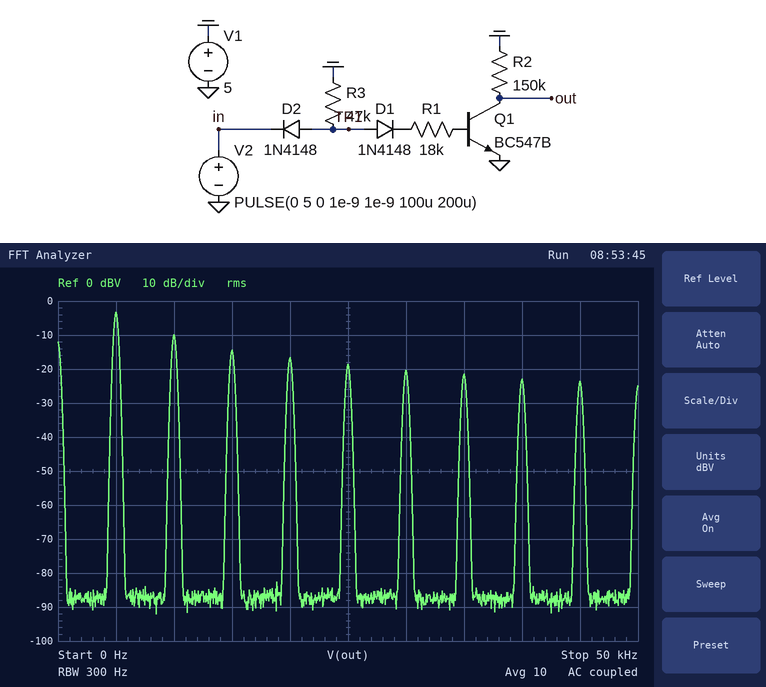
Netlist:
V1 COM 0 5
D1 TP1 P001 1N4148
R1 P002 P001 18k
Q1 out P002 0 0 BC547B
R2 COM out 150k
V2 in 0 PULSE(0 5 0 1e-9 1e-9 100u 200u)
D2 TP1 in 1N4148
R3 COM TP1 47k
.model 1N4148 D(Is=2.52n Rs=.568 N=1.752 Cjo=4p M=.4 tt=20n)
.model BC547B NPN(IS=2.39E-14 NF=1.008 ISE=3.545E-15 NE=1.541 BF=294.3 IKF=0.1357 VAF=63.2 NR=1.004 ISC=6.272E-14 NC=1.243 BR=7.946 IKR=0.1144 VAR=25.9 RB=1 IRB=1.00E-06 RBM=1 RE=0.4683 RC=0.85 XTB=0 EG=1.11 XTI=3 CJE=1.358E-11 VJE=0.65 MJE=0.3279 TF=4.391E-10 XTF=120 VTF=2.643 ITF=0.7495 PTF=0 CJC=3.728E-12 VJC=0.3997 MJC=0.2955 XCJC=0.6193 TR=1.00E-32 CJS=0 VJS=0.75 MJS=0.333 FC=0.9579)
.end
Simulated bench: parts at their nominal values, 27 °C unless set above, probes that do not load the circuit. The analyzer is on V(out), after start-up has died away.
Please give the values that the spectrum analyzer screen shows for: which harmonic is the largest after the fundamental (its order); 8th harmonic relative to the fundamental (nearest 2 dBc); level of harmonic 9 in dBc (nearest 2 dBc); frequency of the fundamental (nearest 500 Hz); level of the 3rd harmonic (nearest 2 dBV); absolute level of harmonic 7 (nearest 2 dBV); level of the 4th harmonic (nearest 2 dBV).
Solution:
2
-20 dBc
-20 dBc
5.0 kHz
-14 dBV
-22 dBV
-16 dBV
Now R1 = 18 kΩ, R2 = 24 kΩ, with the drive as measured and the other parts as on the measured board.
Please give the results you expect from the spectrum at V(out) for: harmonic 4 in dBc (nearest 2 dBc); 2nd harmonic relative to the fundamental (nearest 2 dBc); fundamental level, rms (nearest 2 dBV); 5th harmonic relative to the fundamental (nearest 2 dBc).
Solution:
-16 dBc
-12 dBc
6 dBV
-20 dBc
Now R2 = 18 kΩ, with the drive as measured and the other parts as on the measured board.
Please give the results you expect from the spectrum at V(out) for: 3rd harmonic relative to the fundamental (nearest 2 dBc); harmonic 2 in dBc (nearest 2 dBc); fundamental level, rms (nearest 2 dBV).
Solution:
-12 dBc
-14 dBc
6 dBV
